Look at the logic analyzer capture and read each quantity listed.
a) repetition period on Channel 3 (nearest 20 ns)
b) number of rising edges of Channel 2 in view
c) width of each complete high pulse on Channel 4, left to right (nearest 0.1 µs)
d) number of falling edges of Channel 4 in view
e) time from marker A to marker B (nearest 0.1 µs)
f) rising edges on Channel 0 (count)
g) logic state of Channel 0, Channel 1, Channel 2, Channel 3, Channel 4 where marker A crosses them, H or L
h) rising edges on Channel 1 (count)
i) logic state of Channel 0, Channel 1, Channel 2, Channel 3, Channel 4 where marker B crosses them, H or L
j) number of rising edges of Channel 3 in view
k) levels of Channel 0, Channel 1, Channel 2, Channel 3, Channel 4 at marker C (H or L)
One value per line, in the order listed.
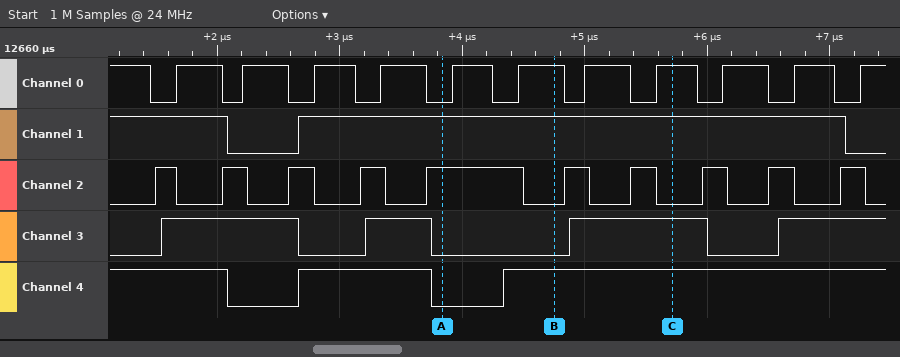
1680 ns
10
1.1 µs
2
0.9 µs
11
Channel 0=L, Channel 1=H, Channel 2=H, Channel 3=L, Channel 4=L
1
Channel 0=H, Channel 1=H, Channel 2=L, Channel 3=L, Channel 4=H
4
Channel 0=H, Channel 1=H, Channel 2=L, Channel 3=H, Channel 4=H
